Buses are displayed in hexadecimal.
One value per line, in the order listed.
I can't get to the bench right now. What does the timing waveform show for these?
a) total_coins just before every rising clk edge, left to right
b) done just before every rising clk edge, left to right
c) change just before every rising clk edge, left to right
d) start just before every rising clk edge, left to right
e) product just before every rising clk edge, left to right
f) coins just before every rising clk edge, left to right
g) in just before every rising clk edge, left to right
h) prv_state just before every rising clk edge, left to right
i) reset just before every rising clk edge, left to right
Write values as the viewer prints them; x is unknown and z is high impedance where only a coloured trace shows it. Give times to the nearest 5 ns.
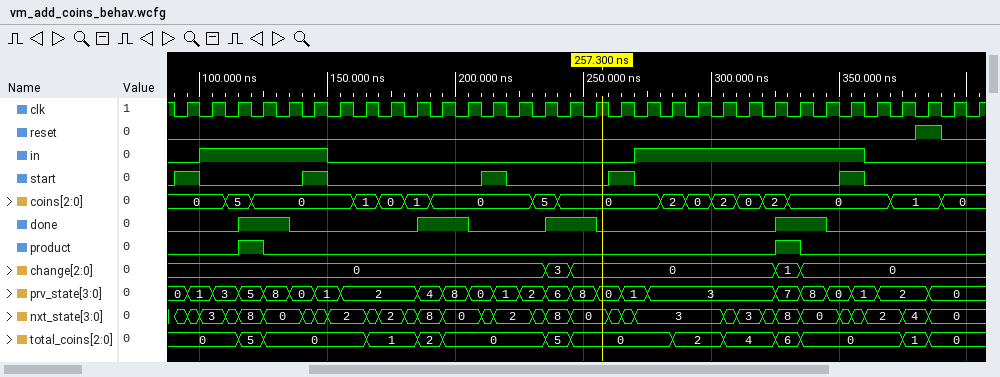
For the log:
0, 0, 0, 5, 0, 0, 0, 0, 1, 1, 2, 0, 0, 0, 0, 5, 0, 0, 0, 0, 2, 2, 4, 4, 6, 0, 0, 0, 0, 1, 0, 0
0 0 0 1 1 0 0 0 0 0 1 1 0 0 0 1 1 0 0 0 0 0 0 0 1 1 0 0 0 0 0 0
0, 0, 0, 0, 0, 0, 0, 0, 0, 0, 0, 0, 0, 0, 0, 3, 0, 0, 0, 0, 0, 0, 0, 0, 1, 0, 0, 0, 0, 0, 0, 0
1 0 0 0 0 1 0 0 0 0 0 0 1 0 0 0 0 1 0 0 0 0 0 0 0 0 1 0 0 0 0 0
0 0 0 1 0 0 0 0 0 0 0 0 0 0 0 0 0 0 0 0 0 0 0 0 1 0 0 0 0 0 0 0
0, 0, 5, 0, 0, 0, 0, 1, 0, 1, 0, 0, 0, 0, 5, 0, 0, 0, 0, 2, 0, 2, 0, 2, 0, 0, 0, 0, 1, 1, 0, 0
0 1 1 1 1 1 0 0 0 0 0 0 0 0 0 0 0 0 1 1 1 1 1 1 1 1 1 0 0 0 0 0
0, 1, 3, 5, 8, 0, 1, 2, 2, 2, 4, 8, 0, 1, 2, 6, 8, 0, 1, 3, 3, 3, 3, 3, 7, 8, 0, 1, 2, 2, 0, 0
0 0 0 0 0 0 0 0 0 0 0 0 0 0 0 0 0 0 0 0 0 0 0 0 0 0 0 0 0 1 0 0
